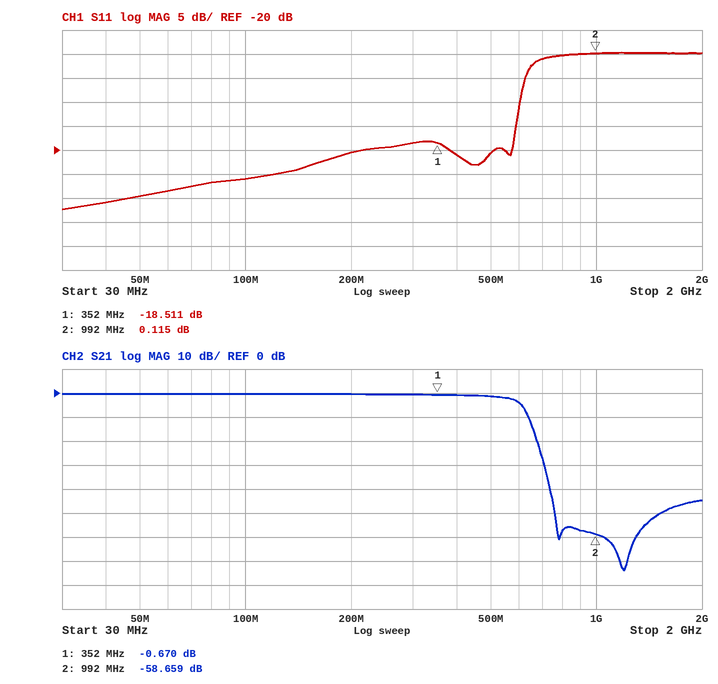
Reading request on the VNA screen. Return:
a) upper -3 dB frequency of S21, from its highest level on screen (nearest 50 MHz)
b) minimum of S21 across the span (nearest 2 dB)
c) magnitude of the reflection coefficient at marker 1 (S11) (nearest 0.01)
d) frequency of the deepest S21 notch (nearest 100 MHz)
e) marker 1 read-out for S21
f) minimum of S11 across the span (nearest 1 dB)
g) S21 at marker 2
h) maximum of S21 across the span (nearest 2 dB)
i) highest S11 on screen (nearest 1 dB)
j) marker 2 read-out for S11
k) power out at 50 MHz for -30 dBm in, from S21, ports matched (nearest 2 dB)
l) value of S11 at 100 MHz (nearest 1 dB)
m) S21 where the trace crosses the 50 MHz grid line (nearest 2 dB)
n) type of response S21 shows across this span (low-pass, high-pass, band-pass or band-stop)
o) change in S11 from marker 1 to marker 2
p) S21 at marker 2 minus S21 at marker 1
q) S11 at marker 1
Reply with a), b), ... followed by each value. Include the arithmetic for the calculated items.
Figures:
a) 600 MHz
b) -74 dB
c) 10^(-18.511/20) ≈ 0.12
d) 1.2 GHz
e) -0.670 dB
f) -32 dB
g) -58.659 dB
h) 0 dB
i) 0 dB
j) 0.115 dB
k) -30 dBm + (0 dB) = -30 dBm
l) -26 dB
m) 0 dB
n) low-pass
o) 0.115 − (-18.511) = 18.626 dB
p) -58.659 − (-0.67) = -57.989 dB
q) -18.511 dB
